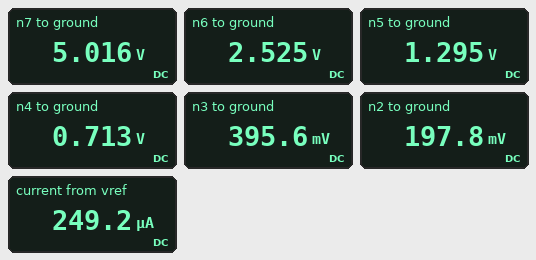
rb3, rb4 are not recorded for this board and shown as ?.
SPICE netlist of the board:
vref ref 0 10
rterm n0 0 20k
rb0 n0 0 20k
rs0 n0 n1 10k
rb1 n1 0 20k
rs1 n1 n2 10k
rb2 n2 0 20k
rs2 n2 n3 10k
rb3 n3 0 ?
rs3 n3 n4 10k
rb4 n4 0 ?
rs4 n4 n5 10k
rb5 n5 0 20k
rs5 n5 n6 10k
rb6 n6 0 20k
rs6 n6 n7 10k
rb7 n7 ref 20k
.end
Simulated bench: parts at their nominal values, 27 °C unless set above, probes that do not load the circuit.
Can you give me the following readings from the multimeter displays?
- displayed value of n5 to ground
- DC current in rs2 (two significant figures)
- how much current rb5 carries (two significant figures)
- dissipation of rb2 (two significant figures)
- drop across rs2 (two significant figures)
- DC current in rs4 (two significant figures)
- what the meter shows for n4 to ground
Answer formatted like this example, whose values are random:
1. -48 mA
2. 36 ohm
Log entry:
1. 1.295 V
2. 20 µA
3. 65 µA
4. 2.0 µW
5. 200 mV
6. 58 µA
7. 0.713 V
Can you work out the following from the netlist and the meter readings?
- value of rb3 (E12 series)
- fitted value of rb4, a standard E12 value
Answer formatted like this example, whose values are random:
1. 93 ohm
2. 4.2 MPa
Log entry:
1. 33 kΩ
2. 27 kΩ
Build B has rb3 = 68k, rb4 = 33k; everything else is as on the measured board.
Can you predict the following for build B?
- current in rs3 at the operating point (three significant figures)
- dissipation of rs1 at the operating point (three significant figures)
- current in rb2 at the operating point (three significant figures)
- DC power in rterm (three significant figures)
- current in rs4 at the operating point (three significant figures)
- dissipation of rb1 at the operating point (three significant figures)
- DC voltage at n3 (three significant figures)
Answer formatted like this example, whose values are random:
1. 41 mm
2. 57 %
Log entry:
1. 30.9 µA
2. 1.42 µW
3. 11.9 µA
4. 178 nW
5. 54.7 µA
6. 711 nW
7. 477 mV
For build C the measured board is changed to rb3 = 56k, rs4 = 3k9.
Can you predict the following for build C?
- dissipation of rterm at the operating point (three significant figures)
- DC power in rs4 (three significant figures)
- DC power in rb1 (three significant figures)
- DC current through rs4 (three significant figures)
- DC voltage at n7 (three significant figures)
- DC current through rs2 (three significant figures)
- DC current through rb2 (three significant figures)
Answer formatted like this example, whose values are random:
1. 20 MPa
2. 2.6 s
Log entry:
1. 225 nW
2. 19.0 µW
3. 901 nW
4. 69.8 µA
5. 4.97 V
6. 26.8 µA
7. 13.4 µA
